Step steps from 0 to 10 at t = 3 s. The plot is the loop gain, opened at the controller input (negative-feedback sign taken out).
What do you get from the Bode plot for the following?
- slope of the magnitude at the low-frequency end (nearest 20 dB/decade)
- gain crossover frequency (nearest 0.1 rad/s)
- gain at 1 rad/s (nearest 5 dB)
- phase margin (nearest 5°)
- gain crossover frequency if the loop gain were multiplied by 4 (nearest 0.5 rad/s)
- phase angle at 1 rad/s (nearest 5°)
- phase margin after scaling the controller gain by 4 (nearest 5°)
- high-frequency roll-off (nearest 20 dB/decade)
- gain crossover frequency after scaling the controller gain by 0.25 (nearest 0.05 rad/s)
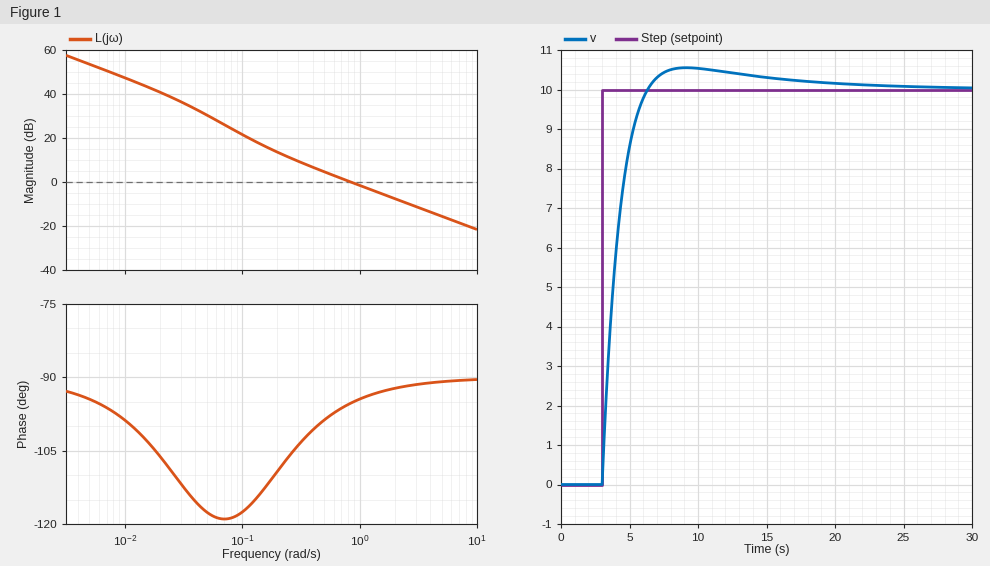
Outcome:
-20 dB/decade
0.8 rad/s
0 dB
85°
3.5 rad/s
-95°
90°
-20 dB/decade
0.25 rad/s
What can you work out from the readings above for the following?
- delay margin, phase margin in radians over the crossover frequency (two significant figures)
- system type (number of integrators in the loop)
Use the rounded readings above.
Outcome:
1.9 s
1
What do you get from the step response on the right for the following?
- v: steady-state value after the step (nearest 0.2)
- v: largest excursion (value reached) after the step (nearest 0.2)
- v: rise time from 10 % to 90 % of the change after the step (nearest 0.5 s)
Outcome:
10.0
10.6
2.0 s
